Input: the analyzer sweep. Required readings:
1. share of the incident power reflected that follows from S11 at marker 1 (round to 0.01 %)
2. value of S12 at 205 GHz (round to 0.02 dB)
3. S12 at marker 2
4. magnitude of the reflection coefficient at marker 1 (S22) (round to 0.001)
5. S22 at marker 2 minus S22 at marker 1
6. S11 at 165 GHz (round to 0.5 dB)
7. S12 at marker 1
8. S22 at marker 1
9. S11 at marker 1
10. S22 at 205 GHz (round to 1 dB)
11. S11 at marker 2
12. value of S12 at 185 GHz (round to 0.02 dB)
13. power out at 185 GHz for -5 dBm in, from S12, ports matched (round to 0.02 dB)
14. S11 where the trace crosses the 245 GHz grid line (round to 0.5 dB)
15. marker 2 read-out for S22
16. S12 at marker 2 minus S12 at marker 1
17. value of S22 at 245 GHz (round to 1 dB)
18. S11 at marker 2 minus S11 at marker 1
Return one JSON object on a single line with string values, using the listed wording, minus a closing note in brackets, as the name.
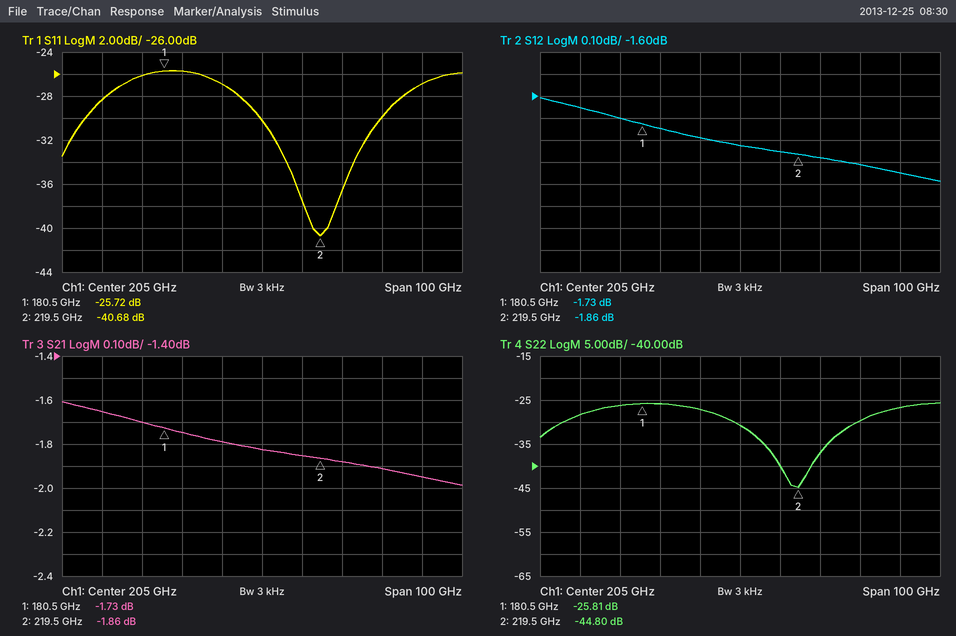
{"share of the incident power reflected that follows from S11 at marker 1": "0.27 %", "value of S12 at 205 GHz": "-1.82 dB", "S12 at marker 2": "-1.86 dB", "magnitude of the reflection coefficient at marker 1 (S22)": "0.051", "S22 at marker 2 minus S22 at marker 1": "-18.99 dB", "S11 at 165 GHz": "-28.5 dB", "S12 at marker 1": "-1.73 dB", "S22 at marker 1": "-25.81 dB", "S11 at marker 1": "-25.72 dB", "S22 at 205 GHz": "-31 dB", "S11 at marker 2": "-40.68 dB", "value of S12 at 185 GHz": "-1.74 dB", "power out at 185 GHz for -5 dBm in, from S12, ports matched": "-6.74 dBm", "S11 where the trace crosses the 245 GHz grid line": "-27.0 dB", "marker 2 read-out for S22": "-44.80 dB", "S12 at marker 2 minus S12 at marker 1": "-0.13 dB", "value of S22 at 245 GHz": "-27 dB", "S11 at marker 2 minus S11 at marker 1": "-14.96 dB"}
